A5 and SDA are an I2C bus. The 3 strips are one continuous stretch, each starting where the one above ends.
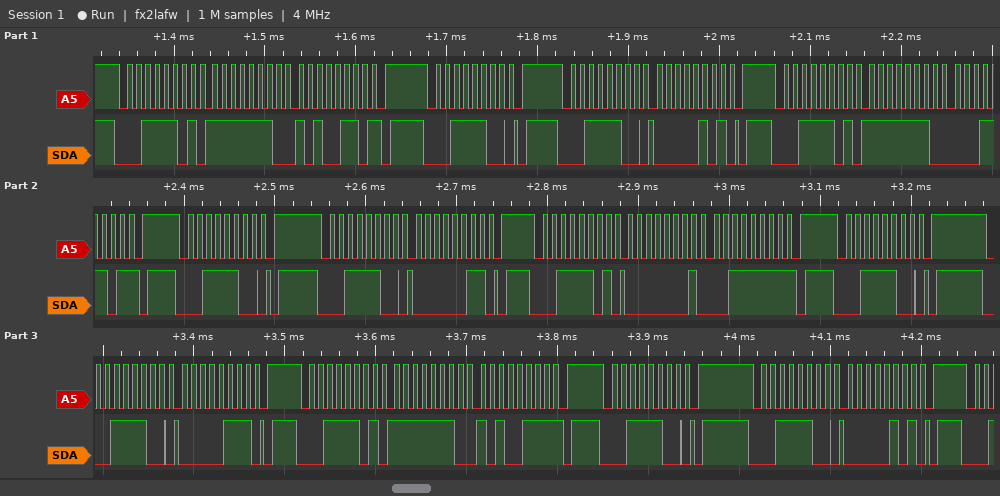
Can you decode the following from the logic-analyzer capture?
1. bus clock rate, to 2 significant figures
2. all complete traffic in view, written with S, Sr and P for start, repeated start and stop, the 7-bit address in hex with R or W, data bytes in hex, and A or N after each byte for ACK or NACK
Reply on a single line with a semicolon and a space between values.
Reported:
100 kHz; S 1ER A FE A A6 N P S 1EW A P S 1EW A 05 A P S 1ER A FE A 1D N P S 1EW A P S 1EW A 03 A P S 1ER A 01 A 3F N P S 1EW A P S 1EW A 07 A P S 1ER A FE A A7 N P S 1EW A P S 1EW A 05 A P
